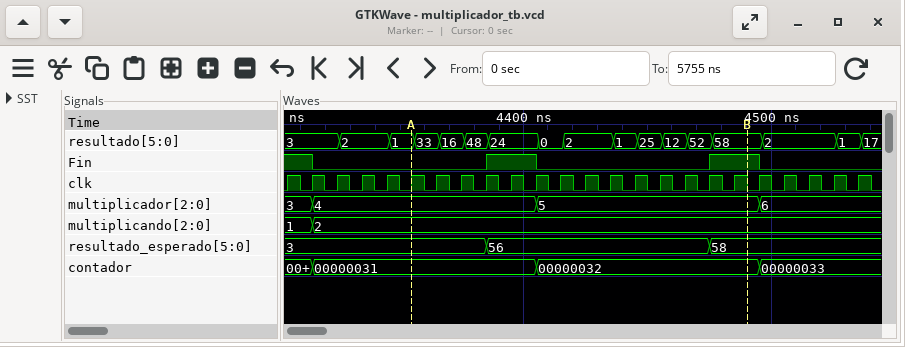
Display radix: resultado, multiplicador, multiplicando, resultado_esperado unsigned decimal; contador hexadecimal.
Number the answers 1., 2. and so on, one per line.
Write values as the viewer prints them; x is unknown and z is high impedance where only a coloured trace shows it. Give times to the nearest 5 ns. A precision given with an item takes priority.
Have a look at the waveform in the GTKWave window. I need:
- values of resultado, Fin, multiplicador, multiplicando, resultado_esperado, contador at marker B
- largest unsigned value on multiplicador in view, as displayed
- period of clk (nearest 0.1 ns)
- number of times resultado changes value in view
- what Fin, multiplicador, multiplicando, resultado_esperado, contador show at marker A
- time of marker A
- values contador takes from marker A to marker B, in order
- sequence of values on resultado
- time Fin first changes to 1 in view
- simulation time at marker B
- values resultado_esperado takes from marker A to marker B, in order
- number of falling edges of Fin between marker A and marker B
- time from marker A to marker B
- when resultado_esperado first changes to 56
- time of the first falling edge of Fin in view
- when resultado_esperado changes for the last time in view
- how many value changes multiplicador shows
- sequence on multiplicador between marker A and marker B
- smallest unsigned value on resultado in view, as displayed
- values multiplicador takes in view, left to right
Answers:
1. resultado=58, Fin=1, multiplicador=5, multiplicando=2, resultado_esperado=58, contador=00000032
2. 6
3. 10 ns
4. 16
5. Fin=0, multiplicador=4, multiplicando=2, resultado_esperado=3, contador=00000031
6. 4355 ns
7. 00000031, 00000032
8. 3, 2, 1, 33, 16, 48, 24, 0, 2, 1, 25, 12, 52, 58, 2, 1, 17
9. 4385 ns
10. 4490 ns
11. 3, 56, 58
12. 1
13. 135 ns
14. 4385 ns
15. 4315 ns
16. 4475 ns
17. 3
18. 4, 5
19. 0
20. 3, 4, 5, 6
